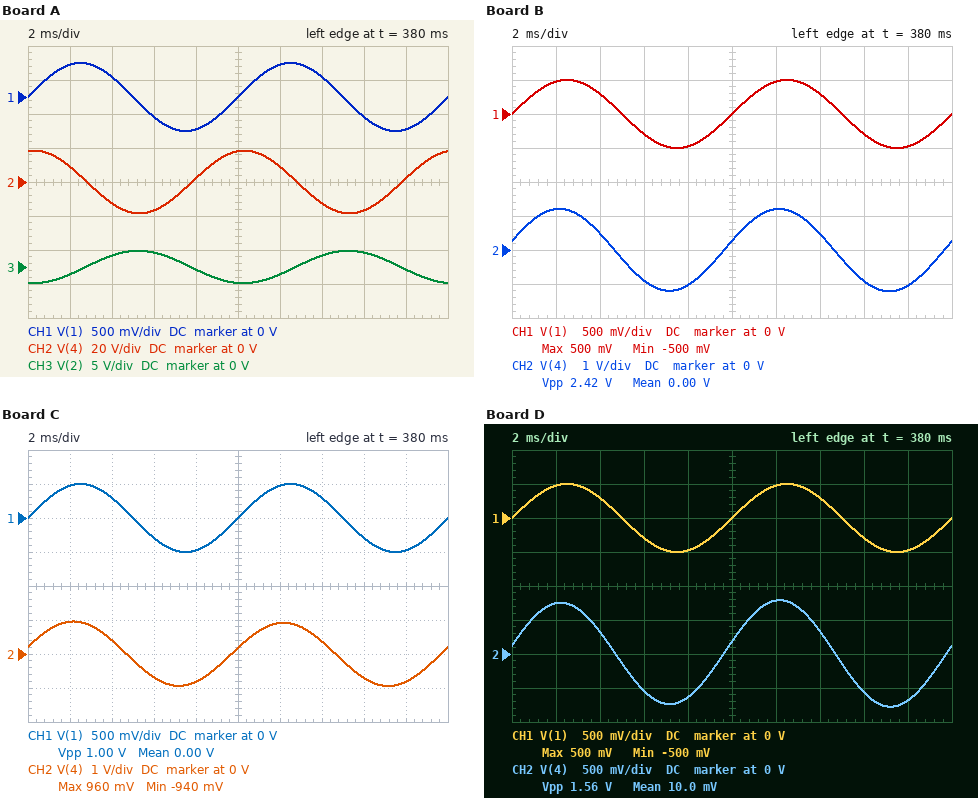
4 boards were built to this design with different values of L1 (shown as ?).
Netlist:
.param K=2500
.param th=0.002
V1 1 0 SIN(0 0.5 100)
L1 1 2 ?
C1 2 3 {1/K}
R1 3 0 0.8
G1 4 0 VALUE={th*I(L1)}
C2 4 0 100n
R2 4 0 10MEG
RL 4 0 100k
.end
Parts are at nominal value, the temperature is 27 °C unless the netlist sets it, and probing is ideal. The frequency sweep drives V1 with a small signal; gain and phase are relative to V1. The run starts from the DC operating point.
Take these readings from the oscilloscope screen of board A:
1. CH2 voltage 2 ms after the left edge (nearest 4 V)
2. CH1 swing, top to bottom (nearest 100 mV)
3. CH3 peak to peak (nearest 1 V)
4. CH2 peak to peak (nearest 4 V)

8 V
1.0 V
5 V
36 V
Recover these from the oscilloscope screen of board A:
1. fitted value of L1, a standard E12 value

6.8 mH
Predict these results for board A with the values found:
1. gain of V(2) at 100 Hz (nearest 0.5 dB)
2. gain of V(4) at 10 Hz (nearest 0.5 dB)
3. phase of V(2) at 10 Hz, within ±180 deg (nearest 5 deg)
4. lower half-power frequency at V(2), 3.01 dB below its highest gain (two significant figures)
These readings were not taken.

13.5 dB
12.5 dB
0 deg
86 Hz
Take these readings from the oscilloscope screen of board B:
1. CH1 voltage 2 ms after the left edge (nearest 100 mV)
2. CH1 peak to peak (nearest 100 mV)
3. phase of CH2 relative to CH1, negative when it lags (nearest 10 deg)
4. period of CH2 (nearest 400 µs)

500 mV
1.0 V
10 deg
10.0 ms
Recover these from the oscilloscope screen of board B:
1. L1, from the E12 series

27 mH
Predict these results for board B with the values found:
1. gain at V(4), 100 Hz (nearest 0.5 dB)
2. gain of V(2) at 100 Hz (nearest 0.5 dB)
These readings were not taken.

7.5 dB
-10.0 dB
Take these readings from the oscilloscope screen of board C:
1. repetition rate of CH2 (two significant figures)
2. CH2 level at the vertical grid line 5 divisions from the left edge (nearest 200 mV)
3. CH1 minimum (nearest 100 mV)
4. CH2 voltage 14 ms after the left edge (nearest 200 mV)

100 Hz
200 mV
-500 mV
400 mV
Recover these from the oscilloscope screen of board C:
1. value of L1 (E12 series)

33 mH
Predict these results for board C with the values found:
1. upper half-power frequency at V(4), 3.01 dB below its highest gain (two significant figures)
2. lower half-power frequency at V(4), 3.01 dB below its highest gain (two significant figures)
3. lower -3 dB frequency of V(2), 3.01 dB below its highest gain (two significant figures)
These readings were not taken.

46 Hz
42 Hz
42 Hz
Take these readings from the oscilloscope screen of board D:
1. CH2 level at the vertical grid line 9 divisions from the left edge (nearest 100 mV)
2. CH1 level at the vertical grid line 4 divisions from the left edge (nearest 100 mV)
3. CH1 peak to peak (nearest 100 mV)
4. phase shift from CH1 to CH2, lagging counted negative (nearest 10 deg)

-700 mV
-500 mV
1.0 V
10 deg
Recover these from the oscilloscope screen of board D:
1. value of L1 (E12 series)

39 mH
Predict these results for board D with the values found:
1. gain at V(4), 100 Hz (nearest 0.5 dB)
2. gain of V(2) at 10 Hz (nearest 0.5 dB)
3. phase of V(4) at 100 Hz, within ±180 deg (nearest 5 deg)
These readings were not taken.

3.5 dB
0.5 dB
10 deg
